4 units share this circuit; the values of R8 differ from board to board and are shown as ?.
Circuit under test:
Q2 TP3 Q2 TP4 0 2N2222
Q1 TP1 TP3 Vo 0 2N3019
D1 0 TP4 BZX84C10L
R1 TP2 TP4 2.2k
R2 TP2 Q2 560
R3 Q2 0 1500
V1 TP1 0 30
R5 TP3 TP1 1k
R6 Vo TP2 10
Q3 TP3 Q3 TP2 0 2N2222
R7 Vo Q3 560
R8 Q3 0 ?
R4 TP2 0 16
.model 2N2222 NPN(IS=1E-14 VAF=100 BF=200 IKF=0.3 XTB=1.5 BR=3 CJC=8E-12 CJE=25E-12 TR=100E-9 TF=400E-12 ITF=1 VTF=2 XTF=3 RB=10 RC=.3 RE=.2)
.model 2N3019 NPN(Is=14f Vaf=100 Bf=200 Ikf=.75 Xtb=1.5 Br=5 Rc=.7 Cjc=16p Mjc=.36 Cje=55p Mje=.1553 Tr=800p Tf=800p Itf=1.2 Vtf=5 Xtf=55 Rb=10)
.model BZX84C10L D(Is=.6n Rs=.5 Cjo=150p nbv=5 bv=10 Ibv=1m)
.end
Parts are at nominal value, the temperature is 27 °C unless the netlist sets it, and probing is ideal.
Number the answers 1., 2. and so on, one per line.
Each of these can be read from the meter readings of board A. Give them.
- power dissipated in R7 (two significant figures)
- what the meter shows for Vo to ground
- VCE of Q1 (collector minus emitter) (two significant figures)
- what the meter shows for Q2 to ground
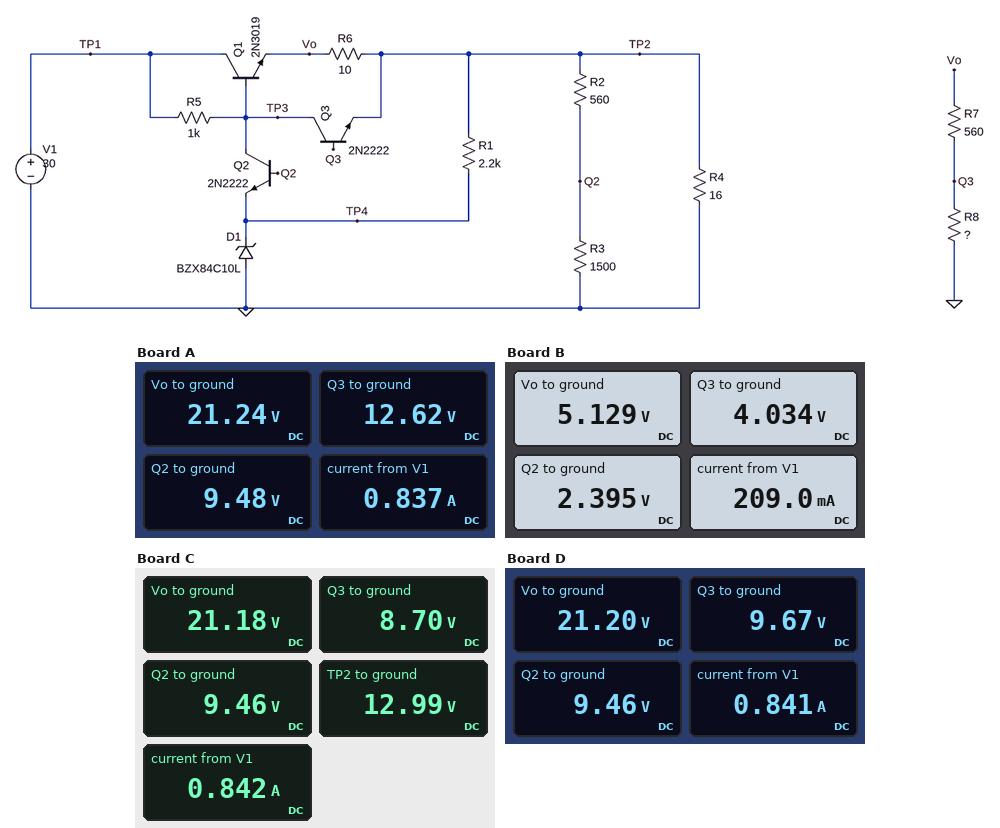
1. 130 mW
2. 21.24 V
3. 8.8 V
4. 9.48 V
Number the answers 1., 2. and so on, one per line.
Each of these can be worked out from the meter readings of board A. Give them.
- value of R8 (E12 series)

1. 820 Ω
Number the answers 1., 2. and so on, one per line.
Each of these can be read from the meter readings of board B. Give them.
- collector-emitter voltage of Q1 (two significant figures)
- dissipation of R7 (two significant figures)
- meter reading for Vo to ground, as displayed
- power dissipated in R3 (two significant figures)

1. 25 V
2. 2.1 mW
3. 5.129 V
4. 3.8 mW
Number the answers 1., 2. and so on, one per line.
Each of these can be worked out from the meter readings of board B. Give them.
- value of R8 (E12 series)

1. 2.2 kΩ
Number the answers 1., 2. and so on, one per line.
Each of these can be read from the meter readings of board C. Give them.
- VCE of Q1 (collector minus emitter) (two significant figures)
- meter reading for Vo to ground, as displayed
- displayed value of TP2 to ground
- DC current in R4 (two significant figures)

1. 8.8 V
2. 21.18 V
3. 12.99 V
4. 810 mA
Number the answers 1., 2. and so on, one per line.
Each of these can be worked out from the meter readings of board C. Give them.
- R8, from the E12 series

1. 390 Ω
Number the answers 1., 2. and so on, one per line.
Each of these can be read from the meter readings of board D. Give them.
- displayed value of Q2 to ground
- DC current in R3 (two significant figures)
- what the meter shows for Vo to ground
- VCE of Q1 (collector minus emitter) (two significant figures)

1. 9.46 V
2. 6.3 mA
3. 21.20 V
4. 8.8 V
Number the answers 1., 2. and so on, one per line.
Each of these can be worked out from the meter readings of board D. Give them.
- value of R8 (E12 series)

1. 470 Ω
